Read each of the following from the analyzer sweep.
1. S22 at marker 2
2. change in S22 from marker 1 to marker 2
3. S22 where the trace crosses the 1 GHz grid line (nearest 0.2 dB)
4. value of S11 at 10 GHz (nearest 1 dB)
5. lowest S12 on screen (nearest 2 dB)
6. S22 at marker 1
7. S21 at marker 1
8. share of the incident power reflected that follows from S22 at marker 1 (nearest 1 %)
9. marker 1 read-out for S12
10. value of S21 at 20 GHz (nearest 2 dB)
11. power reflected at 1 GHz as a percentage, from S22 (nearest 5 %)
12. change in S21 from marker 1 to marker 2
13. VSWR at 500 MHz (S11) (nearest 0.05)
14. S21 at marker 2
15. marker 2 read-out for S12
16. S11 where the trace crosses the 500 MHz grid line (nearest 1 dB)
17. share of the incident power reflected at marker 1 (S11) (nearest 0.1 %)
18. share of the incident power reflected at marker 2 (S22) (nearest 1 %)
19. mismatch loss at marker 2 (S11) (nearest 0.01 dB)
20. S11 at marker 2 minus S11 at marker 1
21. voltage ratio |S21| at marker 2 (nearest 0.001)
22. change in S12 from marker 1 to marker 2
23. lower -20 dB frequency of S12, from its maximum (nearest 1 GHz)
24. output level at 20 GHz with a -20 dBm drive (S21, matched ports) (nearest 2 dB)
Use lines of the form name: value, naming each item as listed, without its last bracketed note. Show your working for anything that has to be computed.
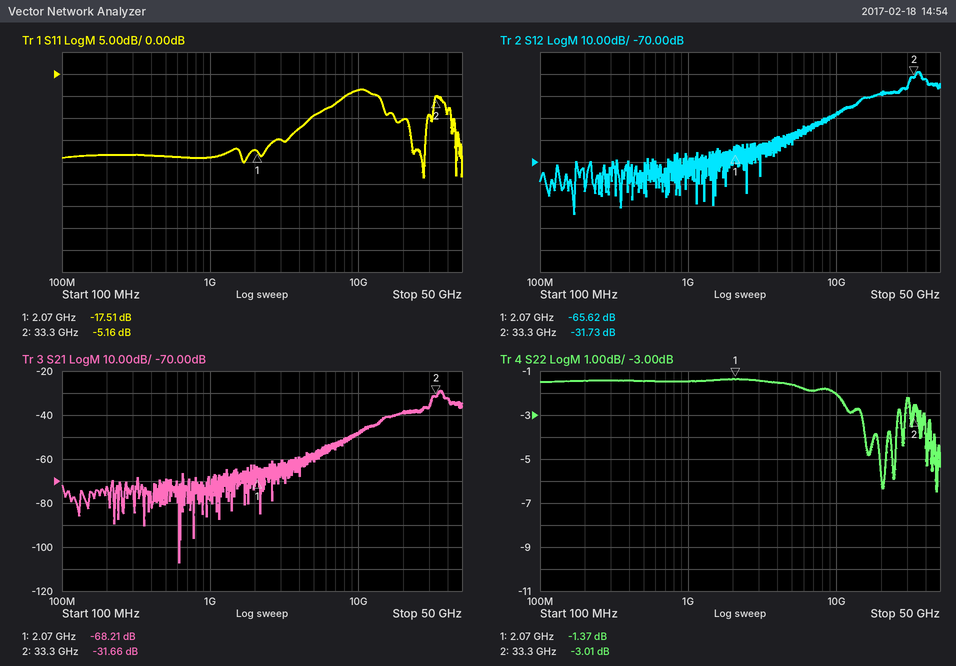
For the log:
S22 at marker 2: -3.01 dB
change in S22 from marker 1 to marker 2: -3.01 − (-1.37) = -1.64 dB
S22 where the trace crosses the 1 GHz grid line: -1.4 dB
value of S11 at 10 GHz: -4 dB
lowest S12 on screen: -94 dB
S22 at marker 1: -1.37 dB
S21 at marker 1: -68.21 dB
share of the incident power reflected that follows from S22 at marker 1: 10^(-1.37/10) ≈ 73 %
marker 1 read-out for S12: -65.62 dB
value of S21 at 20 GHz: -38 dB
power reflected at 1 GHz as a percentage, from S22: 10^(-1.4/10) ≈ 72.4 %, so 70 % to the nearest 5 %
change in S21 from marker 1 to marker 2: -31.66 − (-68.21) = 36.55 dB
VSWR at 500 MHz (S11): |Γ| = 10^(-19/20) = 0.1122; VSWR = (1 + 0.1122)/(1 − 0.1122) ≈ 1.25
S21 at marker 2: -31.66 dB
marker 2 read-out for S12: -31.73 dB
S11 where the trace crosses the 500 MHz grid line: -19 dB
share of the incident power reflected at marker 1 (S11): 10^(-17.51/10) ≈ 1.8 %
share of the incident power reflected at marker 2 (S22): 10^(-3.01/10) ≈ 50 %
mismatch loss at marker 2 (S11): −10 log10(1 − 10^(-5.16/10)) ≈ 1.58 dB
S11 at marker 2 minus S11 at marker 1: -5.16 − (-17.51) = 12.35 dB
voltage ratio |S21| at marker 2: 10^(-31.66/20) ≈ 0.026
change in S12 from marker 1 to marker 2: -31.73 − (-65.62) = 33.89 dB
lower -20 dB frequency of S12, from its maximum: 10 GHz
output level at 20 GHz with a -20 dBm drive (S21, matched ports): -20 dBm + (-38 dB) = -58 dBm
